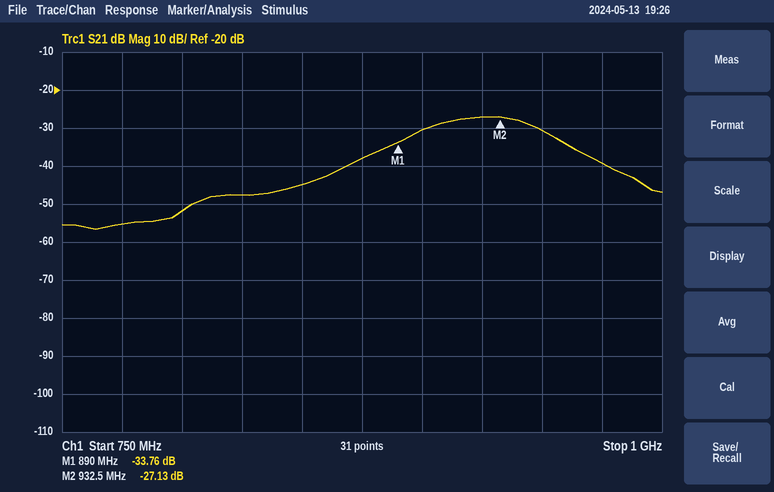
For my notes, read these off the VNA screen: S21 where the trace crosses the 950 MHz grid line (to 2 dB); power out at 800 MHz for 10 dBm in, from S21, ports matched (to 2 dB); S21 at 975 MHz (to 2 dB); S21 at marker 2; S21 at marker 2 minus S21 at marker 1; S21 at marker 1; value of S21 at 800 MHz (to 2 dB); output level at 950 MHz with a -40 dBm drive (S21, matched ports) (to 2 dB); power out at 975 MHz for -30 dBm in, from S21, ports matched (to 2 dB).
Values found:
-30 dB
-42 dBm
-40 dB
-27.13 dB
6.63 dB
-33.76 dB
-52 dB
-70 dBm
-70 dBm
